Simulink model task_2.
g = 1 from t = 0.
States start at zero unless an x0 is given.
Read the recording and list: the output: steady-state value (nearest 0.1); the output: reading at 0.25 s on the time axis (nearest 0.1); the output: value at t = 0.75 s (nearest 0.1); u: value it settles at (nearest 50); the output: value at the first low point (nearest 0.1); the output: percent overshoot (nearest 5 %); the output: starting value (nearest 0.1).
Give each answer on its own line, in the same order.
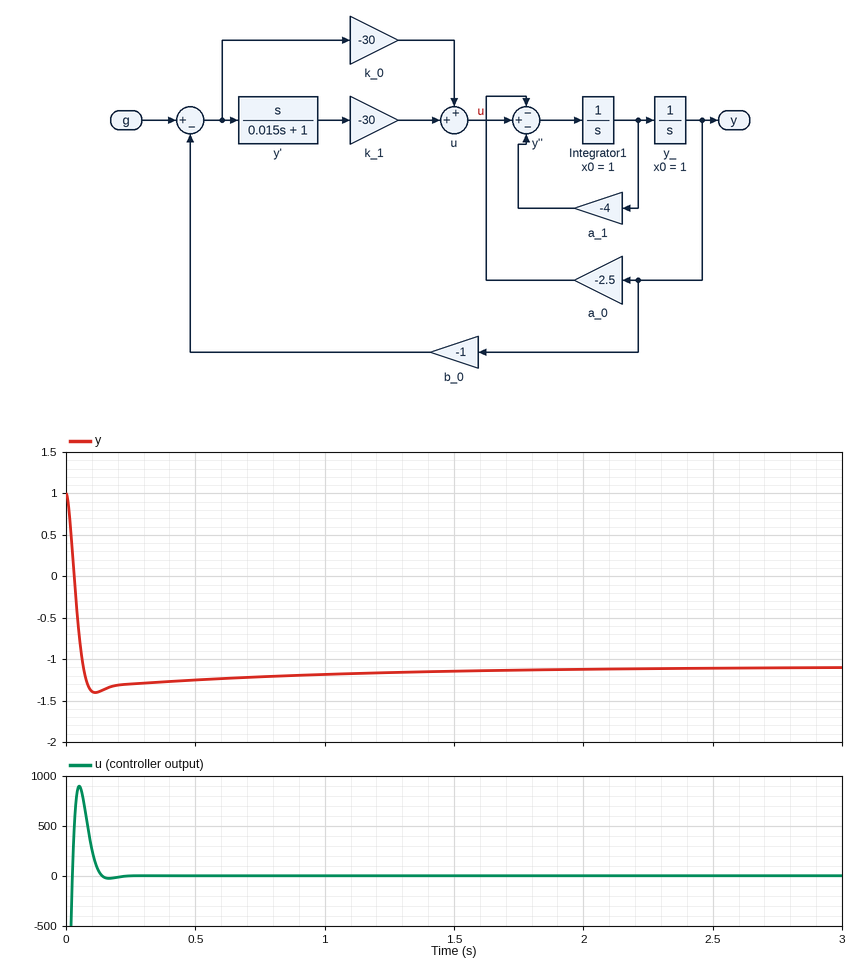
-1.1
-1.3
-1.2
0
-1.4
15 %
1.0
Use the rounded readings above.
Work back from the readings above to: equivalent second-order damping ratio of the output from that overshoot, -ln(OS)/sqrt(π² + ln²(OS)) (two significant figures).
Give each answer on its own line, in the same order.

0.52
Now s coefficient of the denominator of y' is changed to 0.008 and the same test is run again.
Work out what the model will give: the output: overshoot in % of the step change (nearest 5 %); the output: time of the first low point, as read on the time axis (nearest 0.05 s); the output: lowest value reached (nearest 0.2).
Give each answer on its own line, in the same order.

10 %
0.15 s
-1.4
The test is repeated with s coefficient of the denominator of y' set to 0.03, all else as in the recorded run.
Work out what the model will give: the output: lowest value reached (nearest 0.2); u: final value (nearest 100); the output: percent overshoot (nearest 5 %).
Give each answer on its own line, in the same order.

-1.8
0
30 %
